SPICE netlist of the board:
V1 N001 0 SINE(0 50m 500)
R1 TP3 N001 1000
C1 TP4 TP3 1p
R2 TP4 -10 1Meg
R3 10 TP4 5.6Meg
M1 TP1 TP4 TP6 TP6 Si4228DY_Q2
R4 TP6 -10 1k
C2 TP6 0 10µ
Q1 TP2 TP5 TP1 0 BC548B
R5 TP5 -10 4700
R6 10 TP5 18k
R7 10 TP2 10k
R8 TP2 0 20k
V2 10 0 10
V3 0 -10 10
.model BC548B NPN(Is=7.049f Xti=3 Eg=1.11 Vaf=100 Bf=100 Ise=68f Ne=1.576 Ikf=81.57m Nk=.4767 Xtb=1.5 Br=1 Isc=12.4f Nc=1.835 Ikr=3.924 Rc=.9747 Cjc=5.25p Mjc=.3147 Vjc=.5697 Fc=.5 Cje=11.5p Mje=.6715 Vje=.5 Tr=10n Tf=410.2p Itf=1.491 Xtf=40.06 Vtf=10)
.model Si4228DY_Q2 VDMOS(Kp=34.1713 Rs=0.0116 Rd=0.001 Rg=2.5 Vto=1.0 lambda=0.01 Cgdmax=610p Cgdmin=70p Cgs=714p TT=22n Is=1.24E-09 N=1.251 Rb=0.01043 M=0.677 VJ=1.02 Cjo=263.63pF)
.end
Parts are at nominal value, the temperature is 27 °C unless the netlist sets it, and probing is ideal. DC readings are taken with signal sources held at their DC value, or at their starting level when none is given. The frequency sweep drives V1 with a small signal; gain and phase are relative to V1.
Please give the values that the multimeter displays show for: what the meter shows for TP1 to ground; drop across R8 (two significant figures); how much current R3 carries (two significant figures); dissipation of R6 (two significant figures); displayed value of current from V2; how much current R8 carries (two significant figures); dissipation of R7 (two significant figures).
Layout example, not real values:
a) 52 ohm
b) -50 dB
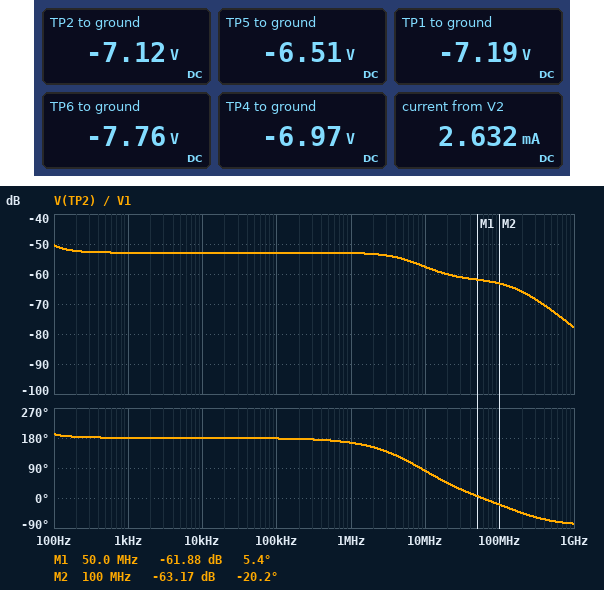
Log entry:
a) -7.19 V
b) 7.1 V
c) 3.0 µA
d) 15 mW
e) 2.632 mA
f) 360 µA
g) 29 mW
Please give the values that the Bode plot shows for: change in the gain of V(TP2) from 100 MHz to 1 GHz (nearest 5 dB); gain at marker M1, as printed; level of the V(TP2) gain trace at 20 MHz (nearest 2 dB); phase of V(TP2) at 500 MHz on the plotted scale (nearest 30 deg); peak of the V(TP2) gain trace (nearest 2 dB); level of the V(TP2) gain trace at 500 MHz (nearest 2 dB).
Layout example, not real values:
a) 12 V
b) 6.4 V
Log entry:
a) -15 dB
b) -61.88 dB
c) -60 dB
d) -60 deg
e) -50 dB
f) -72 dB
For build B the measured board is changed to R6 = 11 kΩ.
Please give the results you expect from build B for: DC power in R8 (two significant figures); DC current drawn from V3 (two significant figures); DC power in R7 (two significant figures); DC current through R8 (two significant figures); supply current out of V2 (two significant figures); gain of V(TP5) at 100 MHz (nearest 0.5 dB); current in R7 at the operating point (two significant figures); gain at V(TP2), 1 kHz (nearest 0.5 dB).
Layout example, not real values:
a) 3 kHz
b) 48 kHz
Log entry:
a) 1.7 mW
b) 3.3 mA
c) 25 mW
d) 290 µA
e) 3.0 mA
f) -63.0 dB
g) 1.6 mA
h) -47.5 dB
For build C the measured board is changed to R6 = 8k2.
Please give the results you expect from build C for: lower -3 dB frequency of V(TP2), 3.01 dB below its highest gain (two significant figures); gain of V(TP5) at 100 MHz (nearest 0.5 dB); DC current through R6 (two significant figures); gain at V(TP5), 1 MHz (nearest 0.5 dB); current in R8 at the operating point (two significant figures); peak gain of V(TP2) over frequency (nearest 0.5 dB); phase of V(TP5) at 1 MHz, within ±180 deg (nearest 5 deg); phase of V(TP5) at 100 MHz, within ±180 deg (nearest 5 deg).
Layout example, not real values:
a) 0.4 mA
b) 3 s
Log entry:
a) 80 Hz
b) -63.0 dB
c) 1.7 mA
d) -45.0 dB
e) 240 µA
f) -36.5 dB
g) 170 deg
h) -5 deg
